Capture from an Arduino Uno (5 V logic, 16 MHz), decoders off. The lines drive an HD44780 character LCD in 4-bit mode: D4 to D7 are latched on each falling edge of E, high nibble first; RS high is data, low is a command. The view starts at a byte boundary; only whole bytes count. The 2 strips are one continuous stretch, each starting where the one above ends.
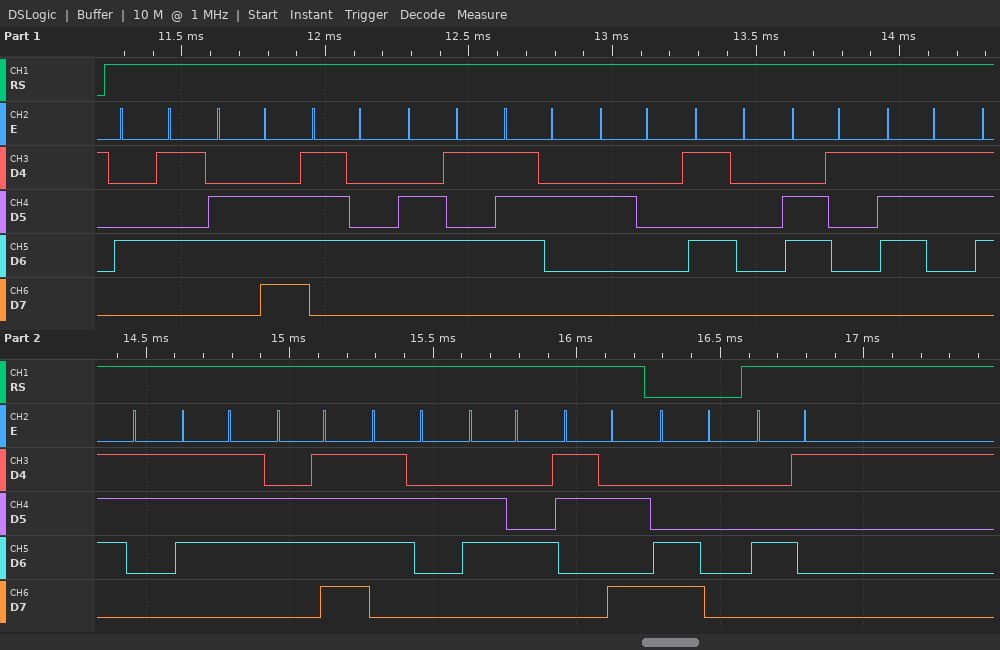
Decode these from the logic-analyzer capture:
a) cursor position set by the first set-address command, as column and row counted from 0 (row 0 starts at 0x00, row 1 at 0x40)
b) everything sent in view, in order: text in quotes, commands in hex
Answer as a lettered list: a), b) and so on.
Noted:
a) column 0, row 1
b) "Enter Password:" 0xC0 "A"
